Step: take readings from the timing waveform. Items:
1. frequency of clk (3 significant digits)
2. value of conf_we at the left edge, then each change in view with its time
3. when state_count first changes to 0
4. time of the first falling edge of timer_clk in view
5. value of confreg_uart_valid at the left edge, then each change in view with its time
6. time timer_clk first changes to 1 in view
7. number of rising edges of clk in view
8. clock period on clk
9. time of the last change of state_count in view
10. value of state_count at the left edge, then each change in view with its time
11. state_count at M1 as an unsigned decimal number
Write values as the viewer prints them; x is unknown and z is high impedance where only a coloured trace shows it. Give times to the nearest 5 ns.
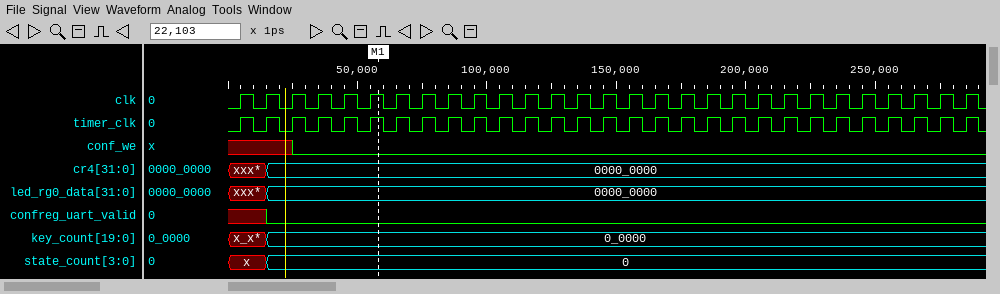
100 MHz
x, 0 at 25 ns
15 ns
10 ns
x, 0 at 15 ns
5 ns
29
10 ns
15 ns
x, 0 at 15 ns
0
